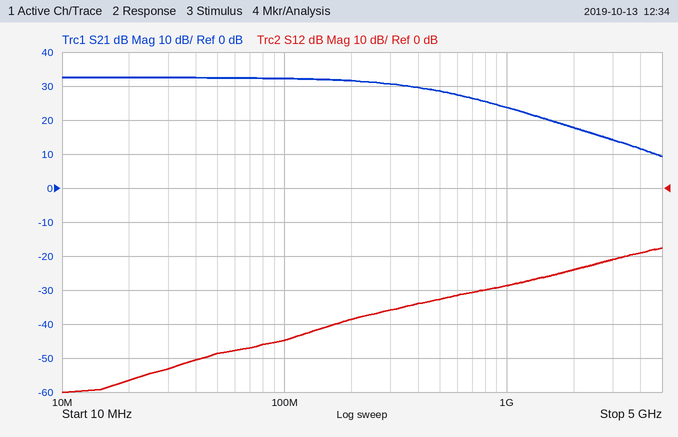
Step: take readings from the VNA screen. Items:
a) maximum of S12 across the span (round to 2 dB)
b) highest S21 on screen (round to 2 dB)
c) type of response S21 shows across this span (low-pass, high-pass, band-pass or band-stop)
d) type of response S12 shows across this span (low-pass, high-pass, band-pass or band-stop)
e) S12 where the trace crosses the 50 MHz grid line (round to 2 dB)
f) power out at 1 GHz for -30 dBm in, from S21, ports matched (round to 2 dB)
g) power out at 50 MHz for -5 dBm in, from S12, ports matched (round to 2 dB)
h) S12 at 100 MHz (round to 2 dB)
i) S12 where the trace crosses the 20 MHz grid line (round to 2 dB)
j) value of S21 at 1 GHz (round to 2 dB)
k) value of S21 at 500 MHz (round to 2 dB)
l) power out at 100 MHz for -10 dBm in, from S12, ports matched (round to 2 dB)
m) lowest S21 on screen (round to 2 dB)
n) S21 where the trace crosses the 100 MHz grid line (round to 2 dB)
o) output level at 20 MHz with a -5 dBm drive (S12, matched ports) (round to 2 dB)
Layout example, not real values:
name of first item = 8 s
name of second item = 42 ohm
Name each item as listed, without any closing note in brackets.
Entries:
maximum of S12 across the span = -18 dB
highest S21 on screen = 32 dB
type of response S21 shows across this span = low-pass
type of response S12 shows across this span = high-pass
S12 where the trace crosses the 50 MHz grid line = -48 dB
power out at 1 GHz for -30 dBm in, from S21, ports matched = -6 dBm
power out at 50 MHz for -5 dBm in, from S12, ports matched = -54 dBm
S12 at 100 MHz = -44 dB
S12 where the trace crosses the 20 MHz grid line = -56 dB
value of S21 at 1 GHz = 24 dB
value of S21 at 500 MHz = 28 dB
power out at 100 MHz for -10 dBm in, from S12, ports matched = -54 dBm
lowest S21 on screen = 10 dB
S21 where the trace crosses the 100 MHz grid line = 32 dB
output level at 20 MHz with a -5 dBm drive (S12, matched ports) = -62 dBm
